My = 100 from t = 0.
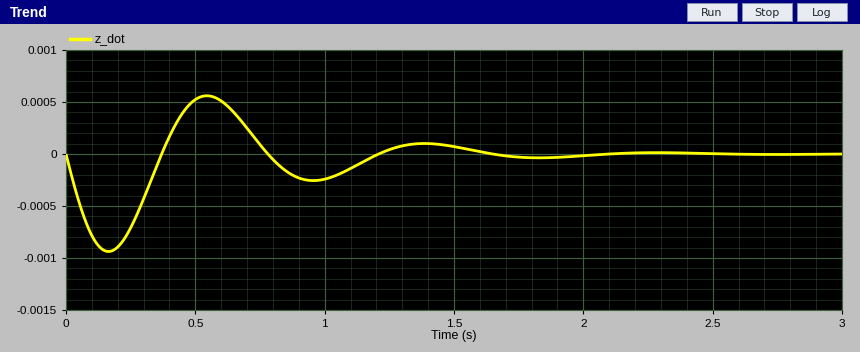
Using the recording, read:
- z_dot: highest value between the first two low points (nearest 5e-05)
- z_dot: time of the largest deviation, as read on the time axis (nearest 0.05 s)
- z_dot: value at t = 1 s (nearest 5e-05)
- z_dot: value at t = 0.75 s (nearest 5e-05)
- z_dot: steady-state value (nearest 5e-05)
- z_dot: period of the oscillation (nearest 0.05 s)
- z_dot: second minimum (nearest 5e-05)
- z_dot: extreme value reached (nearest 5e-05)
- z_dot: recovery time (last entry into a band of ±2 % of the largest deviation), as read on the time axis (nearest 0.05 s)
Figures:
0.00055
0.15 s
-0.00025
0.00010
0.00000
0.80 s
-0.00025
-0.00095
2.00 s
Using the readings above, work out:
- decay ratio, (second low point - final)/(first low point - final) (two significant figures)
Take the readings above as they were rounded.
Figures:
0.26
